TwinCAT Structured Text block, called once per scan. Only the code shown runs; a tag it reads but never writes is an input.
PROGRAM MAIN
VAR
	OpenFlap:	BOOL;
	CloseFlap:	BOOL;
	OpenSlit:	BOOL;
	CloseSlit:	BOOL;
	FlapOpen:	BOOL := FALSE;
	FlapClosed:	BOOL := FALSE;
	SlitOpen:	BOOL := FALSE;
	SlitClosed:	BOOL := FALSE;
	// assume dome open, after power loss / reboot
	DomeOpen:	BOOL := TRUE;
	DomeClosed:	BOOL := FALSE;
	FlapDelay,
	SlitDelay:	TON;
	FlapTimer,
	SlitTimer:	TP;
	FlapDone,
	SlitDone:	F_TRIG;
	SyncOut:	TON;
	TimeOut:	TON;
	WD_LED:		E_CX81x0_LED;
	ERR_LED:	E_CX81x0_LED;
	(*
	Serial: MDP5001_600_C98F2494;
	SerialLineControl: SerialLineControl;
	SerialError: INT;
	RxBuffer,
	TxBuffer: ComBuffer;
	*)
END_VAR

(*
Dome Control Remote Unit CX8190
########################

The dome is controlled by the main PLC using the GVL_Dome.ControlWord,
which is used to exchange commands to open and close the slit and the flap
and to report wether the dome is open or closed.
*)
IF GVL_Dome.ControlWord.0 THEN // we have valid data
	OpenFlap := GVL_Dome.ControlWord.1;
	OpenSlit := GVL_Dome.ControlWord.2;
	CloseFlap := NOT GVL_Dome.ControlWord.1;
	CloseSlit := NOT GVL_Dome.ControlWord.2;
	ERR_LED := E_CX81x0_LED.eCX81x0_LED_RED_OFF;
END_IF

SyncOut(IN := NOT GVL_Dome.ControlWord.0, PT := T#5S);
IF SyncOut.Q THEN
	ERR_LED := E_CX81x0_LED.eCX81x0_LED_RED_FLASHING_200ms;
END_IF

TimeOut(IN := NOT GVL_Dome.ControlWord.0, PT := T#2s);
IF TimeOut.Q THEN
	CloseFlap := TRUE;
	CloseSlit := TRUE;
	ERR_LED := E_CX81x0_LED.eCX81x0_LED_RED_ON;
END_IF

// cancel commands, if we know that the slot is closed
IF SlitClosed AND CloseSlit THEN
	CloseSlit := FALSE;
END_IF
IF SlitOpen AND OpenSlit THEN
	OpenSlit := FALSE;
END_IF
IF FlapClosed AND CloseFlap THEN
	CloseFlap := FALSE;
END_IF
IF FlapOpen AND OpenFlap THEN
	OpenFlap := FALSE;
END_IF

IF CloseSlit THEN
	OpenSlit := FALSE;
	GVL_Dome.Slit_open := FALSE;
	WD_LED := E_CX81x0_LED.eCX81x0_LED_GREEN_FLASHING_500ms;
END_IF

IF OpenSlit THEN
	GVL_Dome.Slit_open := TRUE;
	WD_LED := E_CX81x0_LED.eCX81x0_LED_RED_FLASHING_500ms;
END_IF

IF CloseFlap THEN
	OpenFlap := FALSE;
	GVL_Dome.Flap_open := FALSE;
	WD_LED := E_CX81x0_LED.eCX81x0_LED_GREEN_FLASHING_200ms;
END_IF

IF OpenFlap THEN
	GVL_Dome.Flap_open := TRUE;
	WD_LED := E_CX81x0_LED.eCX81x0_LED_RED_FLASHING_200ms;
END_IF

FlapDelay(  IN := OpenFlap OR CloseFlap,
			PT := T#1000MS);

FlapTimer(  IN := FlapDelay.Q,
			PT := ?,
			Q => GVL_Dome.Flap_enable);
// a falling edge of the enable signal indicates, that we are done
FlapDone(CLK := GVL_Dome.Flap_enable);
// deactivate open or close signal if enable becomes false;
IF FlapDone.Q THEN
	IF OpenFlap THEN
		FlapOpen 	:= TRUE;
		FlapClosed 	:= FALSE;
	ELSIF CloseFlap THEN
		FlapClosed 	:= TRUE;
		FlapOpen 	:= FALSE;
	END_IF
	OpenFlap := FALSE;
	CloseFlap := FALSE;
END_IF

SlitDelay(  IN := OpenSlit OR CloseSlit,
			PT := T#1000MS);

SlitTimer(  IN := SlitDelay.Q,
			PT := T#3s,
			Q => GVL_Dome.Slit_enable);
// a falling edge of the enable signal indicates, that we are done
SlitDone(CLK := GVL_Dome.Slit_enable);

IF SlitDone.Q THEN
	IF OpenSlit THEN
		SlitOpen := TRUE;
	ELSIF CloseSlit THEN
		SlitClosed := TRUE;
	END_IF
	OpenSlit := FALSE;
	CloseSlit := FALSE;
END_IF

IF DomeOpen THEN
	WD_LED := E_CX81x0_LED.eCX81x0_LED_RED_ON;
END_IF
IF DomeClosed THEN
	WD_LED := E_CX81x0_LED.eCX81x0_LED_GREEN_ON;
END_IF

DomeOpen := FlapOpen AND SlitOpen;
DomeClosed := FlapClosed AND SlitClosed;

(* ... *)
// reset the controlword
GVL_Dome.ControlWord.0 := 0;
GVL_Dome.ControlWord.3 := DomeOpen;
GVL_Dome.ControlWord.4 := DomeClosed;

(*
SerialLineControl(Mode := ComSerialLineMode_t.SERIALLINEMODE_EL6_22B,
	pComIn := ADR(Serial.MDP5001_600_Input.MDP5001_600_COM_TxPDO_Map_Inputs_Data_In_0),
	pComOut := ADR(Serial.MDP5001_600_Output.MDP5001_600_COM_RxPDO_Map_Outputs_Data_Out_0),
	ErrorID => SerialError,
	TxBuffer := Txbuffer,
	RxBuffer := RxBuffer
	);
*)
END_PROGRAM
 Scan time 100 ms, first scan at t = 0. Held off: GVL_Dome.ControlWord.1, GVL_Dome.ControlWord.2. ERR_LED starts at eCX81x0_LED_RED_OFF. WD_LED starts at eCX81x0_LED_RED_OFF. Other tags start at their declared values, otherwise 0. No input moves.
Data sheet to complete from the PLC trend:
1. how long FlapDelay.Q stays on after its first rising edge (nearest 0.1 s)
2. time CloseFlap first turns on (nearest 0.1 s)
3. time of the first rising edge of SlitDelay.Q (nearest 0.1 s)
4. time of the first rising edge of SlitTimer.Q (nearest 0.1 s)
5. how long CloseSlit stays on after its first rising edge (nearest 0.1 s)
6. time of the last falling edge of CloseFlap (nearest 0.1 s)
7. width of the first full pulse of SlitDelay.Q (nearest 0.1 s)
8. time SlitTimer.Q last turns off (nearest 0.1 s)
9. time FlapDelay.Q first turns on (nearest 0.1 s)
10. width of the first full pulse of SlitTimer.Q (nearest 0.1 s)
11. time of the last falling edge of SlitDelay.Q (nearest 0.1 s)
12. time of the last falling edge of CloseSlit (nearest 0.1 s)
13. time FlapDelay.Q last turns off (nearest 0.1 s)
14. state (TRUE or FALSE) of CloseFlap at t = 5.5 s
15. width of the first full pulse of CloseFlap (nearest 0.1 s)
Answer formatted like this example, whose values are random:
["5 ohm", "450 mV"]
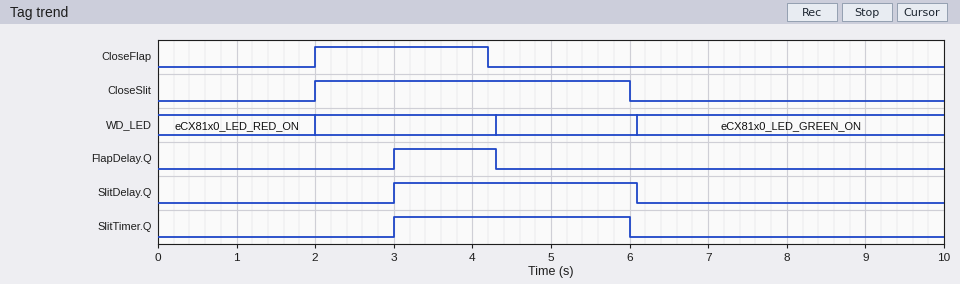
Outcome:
["1.3 s", "2.0 s", "3.0 s", "3.0 s", "4.0 s", "4.2 s", "3.1 s", "6.0 s", "3.0 s", "3.0 s", "6.1 s", "6.0 s", "4.3 s", "FALSE", "2.2 s"]
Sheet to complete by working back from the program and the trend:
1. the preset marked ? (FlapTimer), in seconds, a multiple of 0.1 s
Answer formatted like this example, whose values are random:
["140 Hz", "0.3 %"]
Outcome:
["1.2 s"]
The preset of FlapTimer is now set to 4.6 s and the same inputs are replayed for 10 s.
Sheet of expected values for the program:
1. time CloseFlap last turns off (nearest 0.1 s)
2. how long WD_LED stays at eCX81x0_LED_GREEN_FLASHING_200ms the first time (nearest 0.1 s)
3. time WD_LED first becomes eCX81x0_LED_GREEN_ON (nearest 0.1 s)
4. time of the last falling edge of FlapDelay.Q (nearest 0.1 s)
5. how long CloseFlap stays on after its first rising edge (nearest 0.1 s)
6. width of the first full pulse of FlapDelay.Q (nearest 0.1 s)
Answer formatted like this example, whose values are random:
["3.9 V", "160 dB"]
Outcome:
["7.6 s", "5.7 s", "7.7 s", "7.7 s", "5.6 s", "4.7 s"]
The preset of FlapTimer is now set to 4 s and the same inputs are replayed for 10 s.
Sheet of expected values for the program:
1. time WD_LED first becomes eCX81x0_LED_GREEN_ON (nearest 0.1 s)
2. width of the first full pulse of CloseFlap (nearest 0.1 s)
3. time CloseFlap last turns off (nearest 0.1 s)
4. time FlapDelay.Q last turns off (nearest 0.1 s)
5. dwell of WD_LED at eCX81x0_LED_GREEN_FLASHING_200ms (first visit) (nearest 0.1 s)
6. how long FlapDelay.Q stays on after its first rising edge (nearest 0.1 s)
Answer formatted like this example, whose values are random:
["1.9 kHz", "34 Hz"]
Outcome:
["7.1 s", "5.0 s", "7.0 s", "7.1 s", "5.1 s", "4.1 s"]
